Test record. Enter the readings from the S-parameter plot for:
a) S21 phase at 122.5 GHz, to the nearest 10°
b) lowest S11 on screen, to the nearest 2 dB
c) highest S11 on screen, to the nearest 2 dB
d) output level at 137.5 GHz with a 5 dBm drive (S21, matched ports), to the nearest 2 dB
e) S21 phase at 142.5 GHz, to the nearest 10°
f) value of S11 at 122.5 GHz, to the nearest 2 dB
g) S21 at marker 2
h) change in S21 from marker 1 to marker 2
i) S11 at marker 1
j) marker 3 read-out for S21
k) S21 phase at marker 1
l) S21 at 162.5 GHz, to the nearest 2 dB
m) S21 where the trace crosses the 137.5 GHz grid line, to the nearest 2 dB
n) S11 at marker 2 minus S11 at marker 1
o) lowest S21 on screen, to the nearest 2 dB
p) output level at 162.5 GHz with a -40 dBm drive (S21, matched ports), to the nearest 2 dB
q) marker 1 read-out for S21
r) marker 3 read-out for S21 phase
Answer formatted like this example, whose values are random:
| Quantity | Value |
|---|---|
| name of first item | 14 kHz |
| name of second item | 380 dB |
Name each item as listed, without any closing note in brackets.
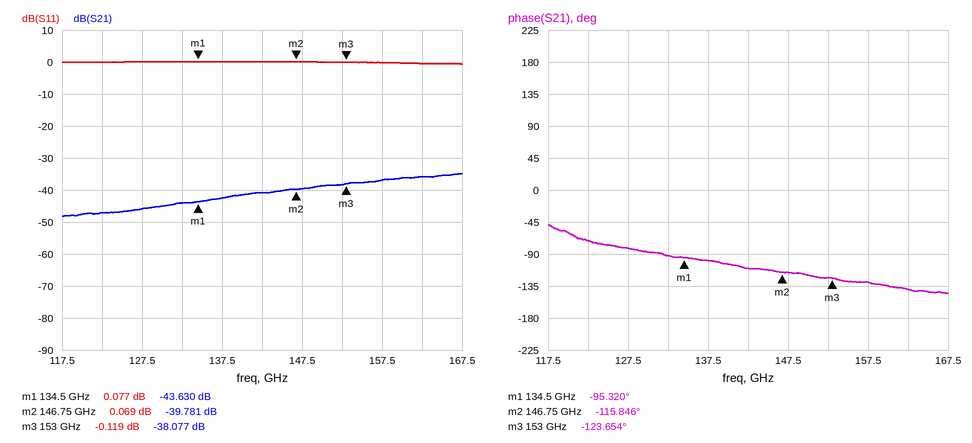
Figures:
| Quantity | Value |
|---|---|
| S21 phase at 122.5 GHz, to the nearest 10° | -70° |
| lowest S11 on screen, to the nearest 2 dB | 0 dB |
| highest S11 on screen, to the nearest 2 dB | 0 dB |
| output level at 137.5 GHz with a 5 dBm drive (S21, matched ports), to the nearest 2 dB | -38 dBm |
| S21 phase at 142.5 GHz, to the nearest 10° | -110° |
| value of S11 at 122.5 GHz, to the nearest 2 dB | 0 dB |
| S21 at marker 2 | -39.781 dB |
| change in S21 from marker 1 to marker 2 | 3.849 dB |
| S11 at marker 1 | 0.077 dB |
| marker 3 read-out for S21 | -38.077 dB |
| S21 phase at marker 1 | -95.320° |
| S21 at 162.5 GHz, to the nearest 2 dB | -36 dB |
| S21 where the trace crosses the 137.5 GHz grid line, to the nearest 2 dB | -42 dB |
| S11 at marker 2 minus S11 at marker 1 | -0.008 dB |
| lowest S21 on screen, to the nearest 2 dB | -48 dB |
| output level at 162.5 GHz with a -40 dBm drive (S21, matched ports), to the nearest 2 dB | -76 dBm |
| marker 1 read-out for S21 | -43.630 dB |
| marker 3 read-out for S21 phase | -123.654° |
